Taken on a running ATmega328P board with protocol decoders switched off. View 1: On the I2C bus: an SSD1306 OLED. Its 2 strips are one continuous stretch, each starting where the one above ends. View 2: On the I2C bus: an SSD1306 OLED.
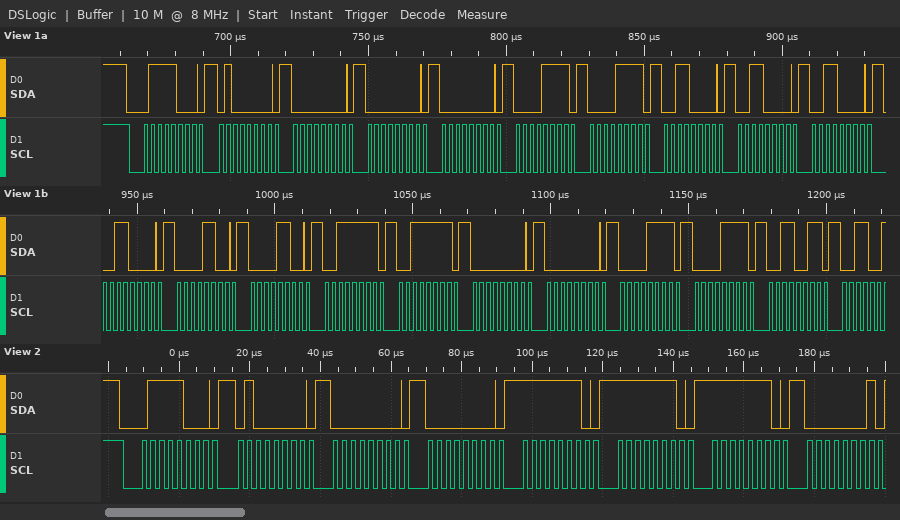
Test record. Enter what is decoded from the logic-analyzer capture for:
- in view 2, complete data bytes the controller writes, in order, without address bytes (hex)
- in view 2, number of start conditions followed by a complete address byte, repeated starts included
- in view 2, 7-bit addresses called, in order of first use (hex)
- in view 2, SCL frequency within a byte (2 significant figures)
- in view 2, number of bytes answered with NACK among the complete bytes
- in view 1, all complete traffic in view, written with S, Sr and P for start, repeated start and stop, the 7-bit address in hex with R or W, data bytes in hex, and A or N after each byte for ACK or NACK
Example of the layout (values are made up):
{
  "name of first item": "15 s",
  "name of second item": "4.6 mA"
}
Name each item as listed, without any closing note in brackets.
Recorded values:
{
  "in view 2, complete data bytes the controller writes, in order, without address bytes": "40 00 00 FE FE FE 01",
  "in view 2, number of start conditions followed by a complete address byte, repeated starts included": "1",
  "in view 2, 7-bit addresses called, in order of first use": "0x3C",
  "in view 2, SCL frequency within a byte": "400 kHz",
  "in view 2, number of bytes answered with NACK among the complete bytes": "0",
  "in view 1, all complete traffic in view, written with S, Sr and P for start, repeated start and stop, the 7-bit address in hex with R or W, data bytes in hex, and A or N after each byte for ACK or NACK": "S 3CW A 40 A 00 A 00 A 00 A 0F A 0F A 30 A 30 A 30 A 30 A 0C A 0C A 3F A 3F A 00 A 00 A 0F A 0F A 33 A"
}
